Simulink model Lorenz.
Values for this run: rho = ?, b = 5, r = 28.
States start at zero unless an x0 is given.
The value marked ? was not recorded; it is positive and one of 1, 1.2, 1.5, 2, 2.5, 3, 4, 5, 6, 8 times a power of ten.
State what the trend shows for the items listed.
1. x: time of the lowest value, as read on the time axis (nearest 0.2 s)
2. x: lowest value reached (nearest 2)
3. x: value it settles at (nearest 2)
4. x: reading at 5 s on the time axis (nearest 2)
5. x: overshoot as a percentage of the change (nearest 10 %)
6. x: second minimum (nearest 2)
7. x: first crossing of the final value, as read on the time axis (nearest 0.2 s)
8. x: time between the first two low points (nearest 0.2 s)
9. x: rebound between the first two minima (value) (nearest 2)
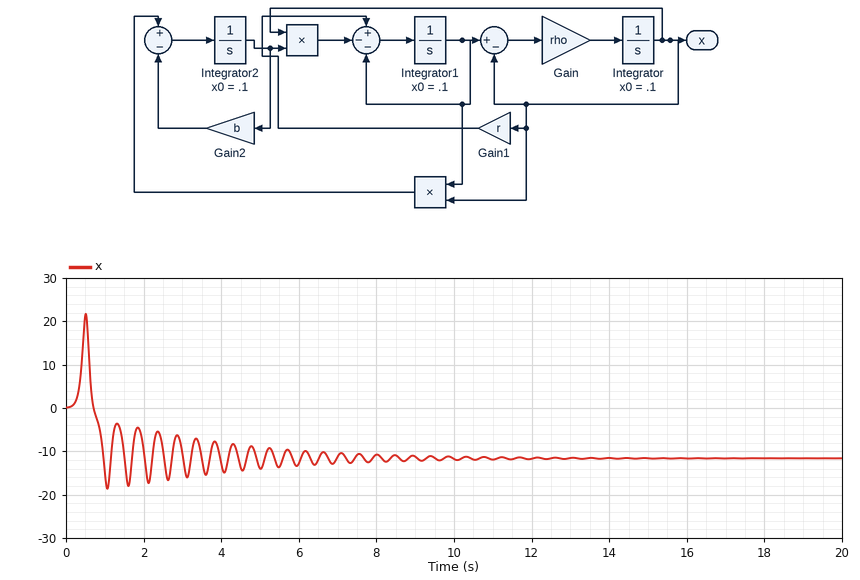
1.0 s
-18
-12
-14
60 %
-18
1.0 s
0.6 s
-4
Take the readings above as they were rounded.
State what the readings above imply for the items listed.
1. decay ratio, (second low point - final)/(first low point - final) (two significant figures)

1.0
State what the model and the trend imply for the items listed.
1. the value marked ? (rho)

12
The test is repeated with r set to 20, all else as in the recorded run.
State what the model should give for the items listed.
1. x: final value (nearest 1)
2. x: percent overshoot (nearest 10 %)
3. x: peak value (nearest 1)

10
70 %
17
